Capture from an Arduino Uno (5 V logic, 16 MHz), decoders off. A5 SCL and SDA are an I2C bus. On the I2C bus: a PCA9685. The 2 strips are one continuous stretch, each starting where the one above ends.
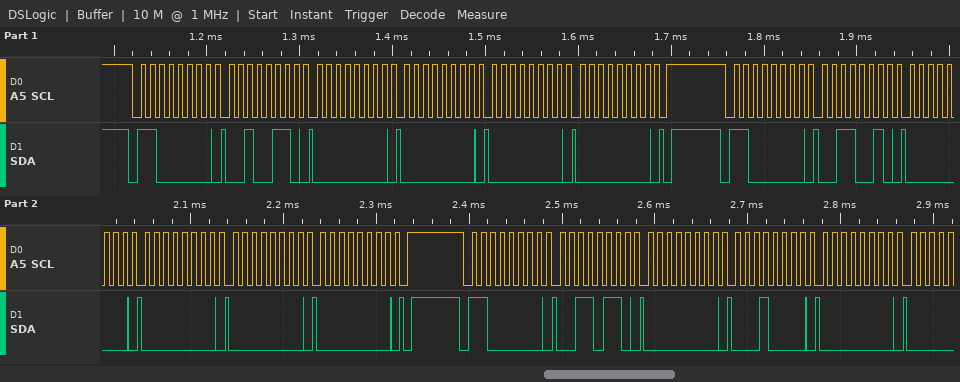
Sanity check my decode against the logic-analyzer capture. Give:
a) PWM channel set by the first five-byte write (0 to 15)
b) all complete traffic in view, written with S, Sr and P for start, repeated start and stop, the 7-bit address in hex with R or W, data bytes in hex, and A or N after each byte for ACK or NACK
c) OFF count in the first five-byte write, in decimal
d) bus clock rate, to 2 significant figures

8
S 60W A 26 A 00 A 00 A 00 A 00 A P S 60W A 32 A 00 A 00 A 00 A 00 A P S 60W A 36 A 00 A 10 A 00 A
0
100 kHz
